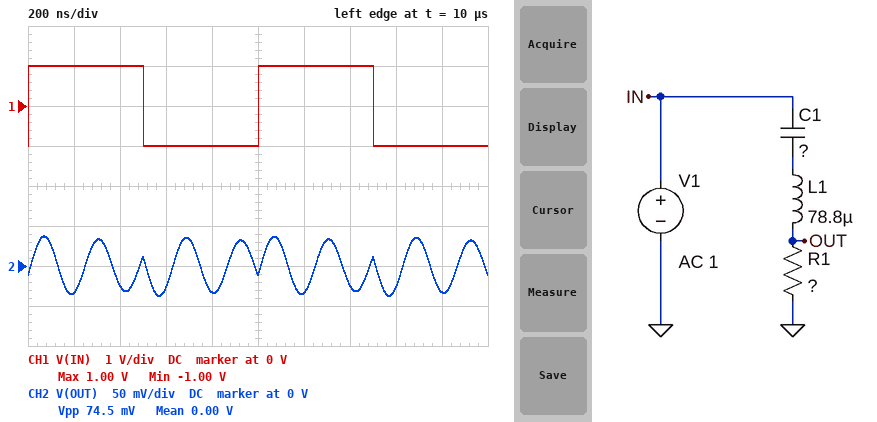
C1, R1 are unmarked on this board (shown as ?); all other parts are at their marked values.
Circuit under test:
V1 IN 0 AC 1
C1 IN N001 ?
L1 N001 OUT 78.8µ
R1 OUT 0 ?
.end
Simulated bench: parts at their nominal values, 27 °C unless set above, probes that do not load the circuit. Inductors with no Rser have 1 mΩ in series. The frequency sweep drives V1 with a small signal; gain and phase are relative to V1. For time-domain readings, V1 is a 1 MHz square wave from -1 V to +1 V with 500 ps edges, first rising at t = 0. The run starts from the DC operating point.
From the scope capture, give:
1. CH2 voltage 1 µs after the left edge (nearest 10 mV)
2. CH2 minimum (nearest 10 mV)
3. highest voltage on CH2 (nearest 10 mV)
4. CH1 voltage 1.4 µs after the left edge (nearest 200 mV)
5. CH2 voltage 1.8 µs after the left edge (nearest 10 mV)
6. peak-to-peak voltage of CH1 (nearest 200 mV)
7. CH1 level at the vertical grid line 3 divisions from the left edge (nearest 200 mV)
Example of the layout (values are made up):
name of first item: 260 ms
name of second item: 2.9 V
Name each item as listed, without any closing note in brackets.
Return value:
CH2 voltage 1 µs after the left edge: -10 mV
CH2 minimum: -40 mV
highest voltage on CH2: 40 mV
CH1 voltage 1.4 µs after the left edge: 1.0 V
CH2 voltage 1.8 µs after the left edge: -30 mV
peak-to-peak voltage of CH1: 2.0 V
CH1 level at the vertical grid line 3 divisions from the left edge: -1.0 V
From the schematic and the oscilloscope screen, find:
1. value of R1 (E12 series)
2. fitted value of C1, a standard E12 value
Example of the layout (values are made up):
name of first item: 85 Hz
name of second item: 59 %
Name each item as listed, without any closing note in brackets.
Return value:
value of R1: 68 Ω
fitted value of C1, a standard E12 value: 18 pF
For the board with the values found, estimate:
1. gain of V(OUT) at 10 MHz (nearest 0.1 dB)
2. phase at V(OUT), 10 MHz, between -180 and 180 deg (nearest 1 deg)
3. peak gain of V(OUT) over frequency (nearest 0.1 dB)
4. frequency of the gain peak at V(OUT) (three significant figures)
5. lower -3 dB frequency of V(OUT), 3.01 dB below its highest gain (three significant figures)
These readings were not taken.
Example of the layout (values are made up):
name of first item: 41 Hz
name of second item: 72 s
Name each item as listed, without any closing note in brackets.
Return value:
gain of V(OUT) at 10 MHz: -35.5 dB
phase at V(OUT), 10 MHz, between -180 and 180 deg: -89 deg
peak gain of V(OUT) over frequency: 0 dB
frequency of the gain peak at V(OUT): 4.23 MHz
lower -3 dB frequency of V(OUT), 3.01 dB below its highest gain: 4.16 MHz
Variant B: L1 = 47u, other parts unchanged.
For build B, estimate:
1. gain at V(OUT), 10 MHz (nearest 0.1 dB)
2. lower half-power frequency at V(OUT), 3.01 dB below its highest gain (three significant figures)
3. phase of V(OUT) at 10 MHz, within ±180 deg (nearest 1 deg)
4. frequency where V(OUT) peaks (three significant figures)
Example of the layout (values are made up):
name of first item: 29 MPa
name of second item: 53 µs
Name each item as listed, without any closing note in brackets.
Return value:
gain at V(OUT), 10 MHz: -29.7 dB
lower half-power frequency at V(OUT), 3.01 dB below its highest gain: 5.36 MHz
phase of V(OUT) at 10 MHz, within ±180 deg: -88 deg
frequency where V(OUT) peaks: 5.47 MHz
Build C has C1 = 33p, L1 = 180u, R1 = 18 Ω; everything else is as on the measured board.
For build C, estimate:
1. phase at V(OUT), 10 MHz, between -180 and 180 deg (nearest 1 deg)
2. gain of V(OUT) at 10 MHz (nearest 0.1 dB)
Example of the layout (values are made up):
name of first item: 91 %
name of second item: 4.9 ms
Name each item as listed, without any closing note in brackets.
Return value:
phase at V(OUT), 10 MHz, between -180 and 180 deg: -90 deg
gain of V(OUT) at 10 MHz: -55.6 dB
